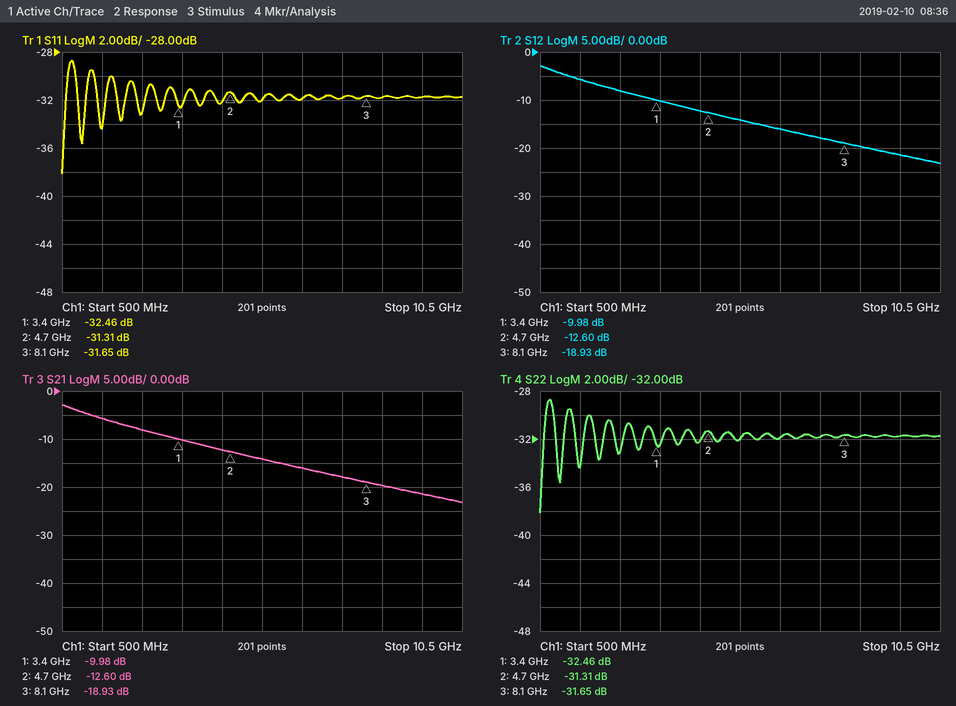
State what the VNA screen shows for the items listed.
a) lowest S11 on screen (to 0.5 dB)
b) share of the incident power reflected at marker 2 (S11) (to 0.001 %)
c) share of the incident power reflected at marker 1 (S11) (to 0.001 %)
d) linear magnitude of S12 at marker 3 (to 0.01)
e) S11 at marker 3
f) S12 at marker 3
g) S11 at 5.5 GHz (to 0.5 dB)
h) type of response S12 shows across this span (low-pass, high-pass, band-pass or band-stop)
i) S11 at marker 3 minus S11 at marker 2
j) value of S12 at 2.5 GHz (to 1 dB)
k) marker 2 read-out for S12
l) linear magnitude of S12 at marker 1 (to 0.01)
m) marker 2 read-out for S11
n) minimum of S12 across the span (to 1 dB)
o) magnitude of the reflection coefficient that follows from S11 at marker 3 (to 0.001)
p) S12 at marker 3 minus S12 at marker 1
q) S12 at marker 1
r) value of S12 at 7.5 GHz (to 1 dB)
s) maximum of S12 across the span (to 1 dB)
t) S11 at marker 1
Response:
-38.0 dB
0.074 %
0.057 %
0.11
-31.65 dB
-18.93 dB
-32.0 dB
low-pass
-0.34 dB
-8 dB
-12.60 dB
0.32
-31.31 dB
-23 dB
0.026
-8.95 dB
-9.98 dB
-18 dB
-3 dB
-32.46 dB
